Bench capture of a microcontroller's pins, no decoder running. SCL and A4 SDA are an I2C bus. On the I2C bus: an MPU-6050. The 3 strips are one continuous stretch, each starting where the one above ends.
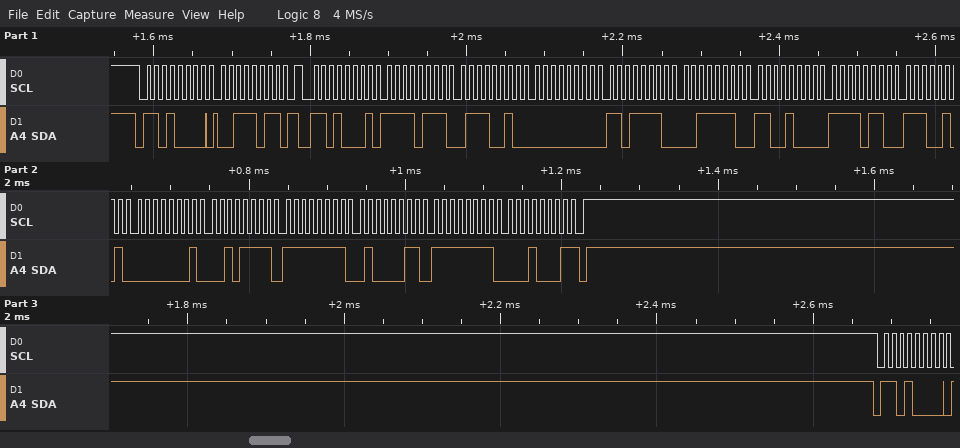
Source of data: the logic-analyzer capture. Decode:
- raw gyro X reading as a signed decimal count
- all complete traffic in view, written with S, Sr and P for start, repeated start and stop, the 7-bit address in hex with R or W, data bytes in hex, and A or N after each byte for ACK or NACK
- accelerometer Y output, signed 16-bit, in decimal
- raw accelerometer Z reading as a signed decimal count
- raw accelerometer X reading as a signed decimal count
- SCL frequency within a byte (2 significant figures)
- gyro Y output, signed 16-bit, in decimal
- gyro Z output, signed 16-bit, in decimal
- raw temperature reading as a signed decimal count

303
S 68W A 3B A Sr 68R A F7 A 72 A 00 A DE A 3E A C8 A F6 A E5 A 01 A 2F A FF A 43 A FF A 11 N P S 68W A
222
16072
-2190
100 kHz
-189
-239
-2331
